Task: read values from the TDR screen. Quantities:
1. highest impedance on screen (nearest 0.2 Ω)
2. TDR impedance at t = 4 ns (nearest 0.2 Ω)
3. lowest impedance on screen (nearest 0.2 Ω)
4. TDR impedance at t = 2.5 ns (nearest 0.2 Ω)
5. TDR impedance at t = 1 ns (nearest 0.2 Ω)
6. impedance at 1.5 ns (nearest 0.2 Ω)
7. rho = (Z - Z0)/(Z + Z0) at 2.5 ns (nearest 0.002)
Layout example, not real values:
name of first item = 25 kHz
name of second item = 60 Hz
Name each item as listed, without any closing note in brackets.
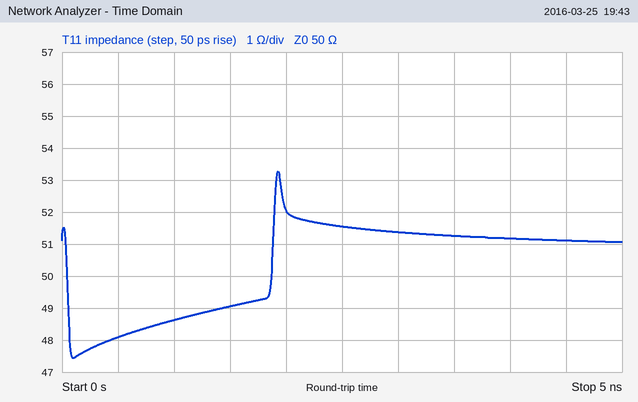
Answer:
highest impedance on screen = 53.2 Ω
TDR impedance at t = 4 ns = 51.2 Ω
lowest impedance on screen = 47.4 Ω
TDR impedance at t = 2.5 ns = 51.6 Ω
TDR impedance at t = 1 ns = 48.6 Ω
impedance at 1.5 ns = 49.0 Ω
rho = (Z - Z0)/(Z + Z0) at 2.5 ns = +0.016
